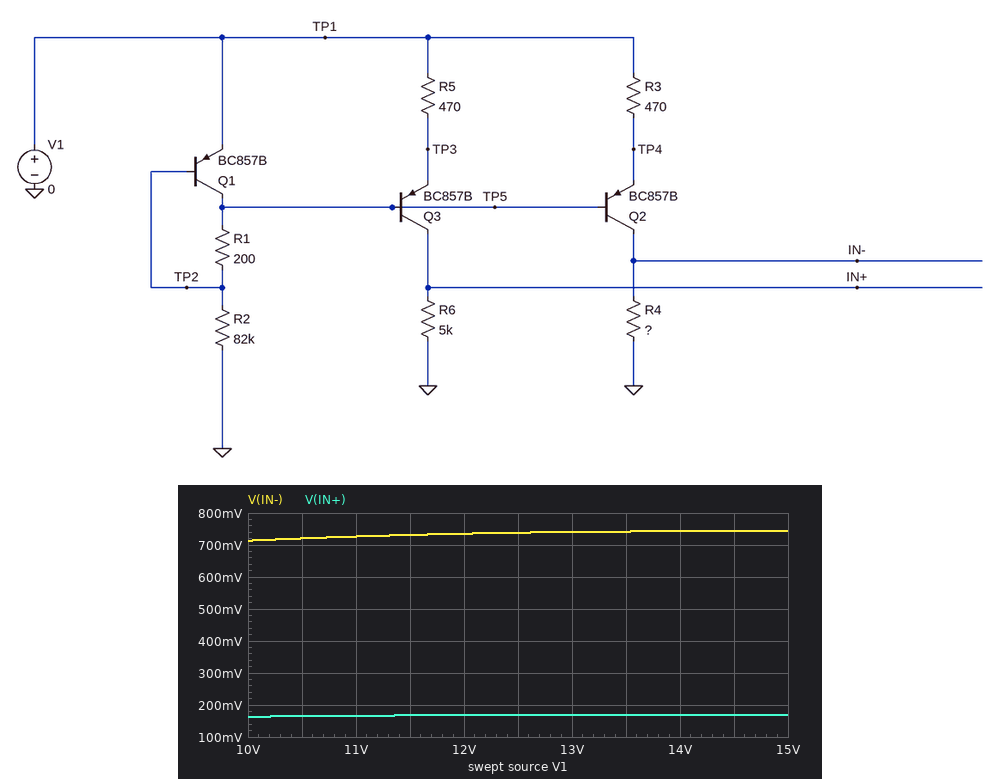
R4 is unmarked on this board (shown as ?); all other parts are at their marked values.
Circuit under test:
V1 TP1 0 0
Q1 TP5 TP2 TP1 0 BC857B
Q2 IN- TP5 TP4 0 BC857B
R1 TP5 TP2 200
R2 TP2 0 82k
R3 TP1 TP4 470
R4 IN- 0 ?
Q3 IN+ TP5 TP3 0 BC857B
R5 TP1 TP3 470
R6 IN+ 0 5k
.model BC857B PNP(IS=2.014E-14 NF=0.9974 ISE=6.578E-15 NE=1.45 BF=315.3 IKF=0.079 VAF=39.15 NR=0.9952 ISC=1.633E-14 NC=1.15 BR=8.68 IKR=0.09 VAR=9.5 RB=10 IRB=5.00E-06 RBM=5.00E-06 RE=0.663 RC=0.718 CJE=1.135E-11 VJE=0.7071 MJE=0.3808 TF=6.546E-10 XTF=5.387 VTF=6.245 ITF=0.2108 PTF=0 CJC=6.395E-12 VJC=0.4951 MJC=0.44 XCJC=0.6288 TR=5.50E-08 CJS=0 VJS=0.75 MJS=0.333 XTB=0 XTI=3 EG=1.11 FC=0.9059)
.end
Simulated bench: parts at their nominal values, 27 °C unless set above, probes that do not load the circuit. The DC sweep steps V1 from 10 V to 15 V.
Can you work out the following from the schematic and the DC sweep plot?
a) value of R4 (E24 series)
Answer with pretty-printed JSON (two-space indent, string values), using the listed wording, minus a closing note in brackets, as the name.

{
  "value of R4": "22 kΩ"
}
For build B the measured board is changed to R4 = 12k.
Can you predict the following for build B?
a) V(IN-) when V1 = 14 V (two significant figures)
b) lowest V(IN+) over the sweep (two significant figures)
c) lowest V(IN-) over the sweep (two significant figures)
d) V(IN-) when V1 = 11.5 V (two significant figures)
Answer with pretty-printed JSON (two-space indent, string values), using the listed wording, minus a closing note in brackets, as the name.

{
  "V(IN-) when V1 = 14 V": "410 mV",
  "lowest V(IN+) over the sweep": "160 mV",
  "lowest V(IN-) over the sweep": "390 mV",
  "V(IN-) when V1 = 11.5 V": "400 mV"
}
